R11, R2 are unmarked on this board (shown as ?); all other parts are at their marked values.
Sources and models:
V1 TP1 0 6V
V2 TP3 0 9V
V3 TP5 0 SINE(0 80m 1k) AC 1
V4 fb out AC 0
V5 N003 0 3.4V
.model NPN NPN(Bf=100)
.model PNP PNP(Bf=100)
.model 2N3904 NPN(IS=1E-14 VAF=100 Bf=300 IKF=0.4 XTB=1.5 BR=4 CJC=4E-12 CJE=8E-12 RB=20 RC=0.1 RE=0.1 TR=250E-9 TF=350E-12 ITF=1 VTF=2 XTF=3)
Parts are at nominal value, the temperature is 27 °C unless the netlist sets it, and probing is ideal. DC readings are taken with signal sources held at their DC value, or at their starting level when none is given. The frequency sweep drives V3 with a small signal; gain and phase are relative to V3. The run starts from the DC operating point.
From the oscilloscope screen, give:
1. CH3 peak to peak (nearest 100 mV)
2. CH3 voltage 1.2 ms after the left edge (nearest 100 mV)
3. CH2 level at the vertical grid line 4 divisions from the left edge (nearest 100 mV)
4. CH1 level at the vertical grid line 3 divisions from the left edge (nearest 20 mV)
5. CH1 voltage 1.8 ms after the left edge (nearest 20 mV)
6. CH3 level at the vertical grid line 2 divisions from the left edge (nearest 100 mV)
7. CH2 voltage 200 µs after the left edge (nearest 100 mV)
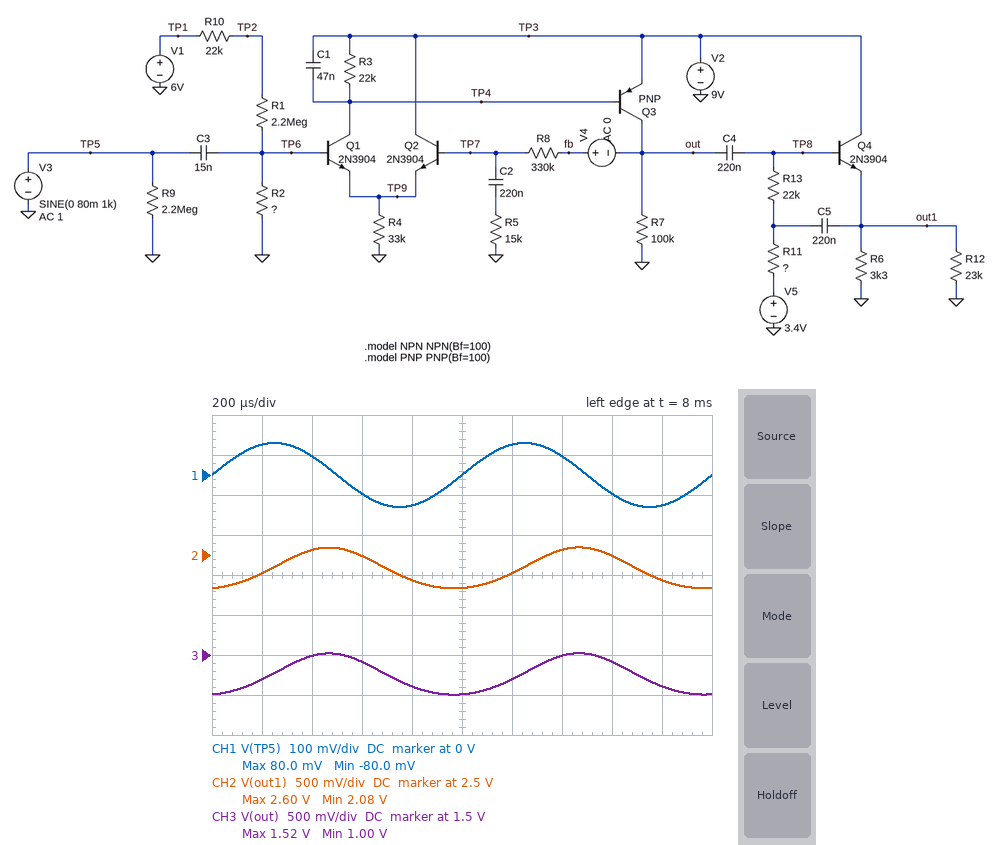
500 mV
1.2 V
2.2 V
-40 mV
-80 mV
1.5 V
2.3 V
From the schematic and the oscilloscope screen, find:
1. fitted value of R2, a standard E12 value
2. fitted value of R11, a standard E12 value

820 kΩ
150 kΩ
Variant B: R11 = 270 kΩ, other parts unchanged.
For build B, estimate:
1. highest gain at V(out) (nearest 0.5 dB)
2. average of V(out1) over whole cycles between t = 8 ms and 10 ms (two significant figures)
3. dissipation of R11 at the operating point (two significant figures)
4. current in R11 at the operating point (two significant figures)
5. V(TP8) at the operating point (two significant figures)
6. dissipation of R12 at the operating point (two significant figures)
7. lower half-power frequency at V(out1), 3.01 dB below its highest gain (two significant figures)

24.5 dB
2.1 V
1.4 µW
2.3 µA
2.7 V
190 µW
18 Hz
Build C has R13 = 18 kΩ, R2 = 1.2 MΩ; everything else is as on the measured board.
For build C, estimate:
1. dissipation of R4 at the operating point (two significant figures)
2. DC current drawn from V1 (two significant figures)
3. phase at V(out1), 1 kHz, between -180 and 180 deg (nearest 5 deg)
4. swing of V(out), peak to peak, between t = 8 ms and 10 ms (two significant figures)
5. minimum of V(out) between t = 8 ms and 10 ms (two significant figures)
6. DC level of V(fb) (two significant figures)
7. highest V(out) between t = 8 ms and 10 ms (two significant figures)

65 µW
1.8 µA
-15 deg
3.2 V
810 mV
2.0 V
4.0 V
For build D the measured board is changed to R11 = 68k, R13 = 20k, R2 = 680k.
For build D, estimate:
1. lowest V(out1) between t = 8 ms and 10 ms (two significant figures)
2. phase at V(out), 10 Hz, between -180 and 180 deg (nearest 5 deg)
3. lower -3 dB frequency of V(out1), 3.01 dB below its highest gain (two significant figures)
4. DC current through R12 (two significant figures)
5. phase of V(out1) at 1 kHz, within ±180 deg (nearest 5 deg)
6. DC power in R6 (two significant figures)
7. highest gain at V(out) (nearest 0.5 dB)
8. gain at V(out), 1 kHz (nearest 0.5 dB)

2.5 V
45 deg
28 Hz
110 µA
-80 deg
1.9 mW
-18.0 dB
-31.0 dB
